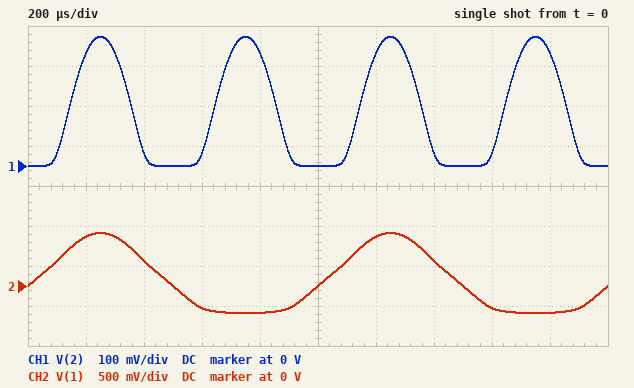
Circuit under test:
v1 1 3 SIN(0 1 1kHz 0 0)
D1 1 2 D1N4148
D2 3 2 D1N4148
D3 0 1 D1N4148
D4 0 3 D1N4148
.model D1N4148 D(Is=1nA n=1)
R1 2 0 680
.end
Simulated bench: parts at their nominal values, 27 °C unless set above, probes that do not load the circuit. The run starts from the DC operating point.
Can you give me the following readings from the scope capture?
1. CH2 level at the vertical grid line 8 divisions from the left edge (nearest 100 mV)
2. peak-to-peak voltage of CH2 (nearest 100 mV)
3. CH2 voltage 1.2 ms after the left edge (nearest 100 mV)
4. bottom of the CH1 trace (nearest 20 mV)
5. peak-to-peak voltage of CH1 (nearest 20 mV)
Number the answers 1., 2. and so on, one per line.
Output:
1. -300 mV
2. 1.0 V
3. 600 mV
4. 0 V
5. 320 mV
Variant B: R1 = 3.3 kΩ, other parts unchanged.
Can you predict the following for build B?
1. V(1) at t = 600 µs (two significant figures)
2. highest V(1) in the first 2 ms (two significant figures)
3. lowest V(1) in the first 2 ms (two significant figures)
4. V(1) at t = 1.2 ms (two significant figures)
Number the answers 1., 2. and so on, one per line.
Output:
1. -260 mV
2. 700 mV
3. -300 mV
4. 650 mV
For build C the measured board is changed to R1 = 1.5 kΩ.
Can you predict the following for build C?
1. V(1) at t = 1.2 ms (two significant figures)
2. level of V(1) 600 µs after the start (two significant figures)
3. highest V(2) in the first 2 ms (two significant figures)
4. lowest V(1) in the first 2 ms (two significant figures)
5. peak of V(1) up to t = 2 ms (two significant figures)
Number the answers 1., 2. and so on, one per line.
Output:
1. 630 mV
2. -270 mV
3. 360 mV
4. -320 mV
5. 680 mV
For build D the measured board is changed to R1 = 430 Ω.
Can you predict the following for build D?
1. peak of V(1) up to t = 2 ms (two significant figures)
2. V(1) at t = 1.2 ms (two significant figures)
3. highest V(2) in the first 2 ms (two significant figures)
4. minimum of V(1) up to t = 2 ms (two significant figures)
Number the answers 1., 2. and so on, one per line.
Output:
1. 650 mV
2. 610 mV
3. 300 mV
4. -350 mV
